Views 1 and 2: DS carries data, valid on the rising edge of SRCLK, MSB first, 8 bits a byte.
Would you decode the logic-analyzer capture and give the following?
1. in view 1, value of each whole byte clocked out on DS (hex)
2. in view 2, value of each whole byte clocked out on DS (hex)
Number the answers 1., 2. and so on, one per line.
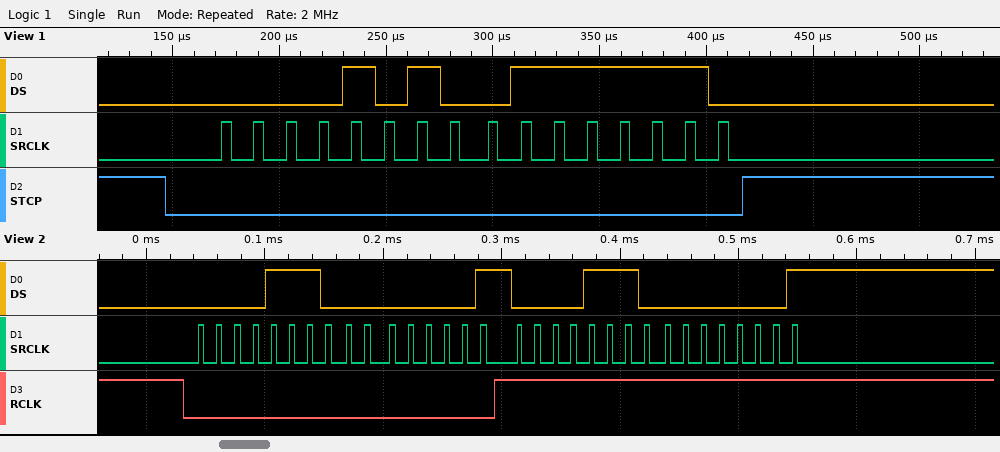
1. 0A 7E
2. 0E 01 0E 01
